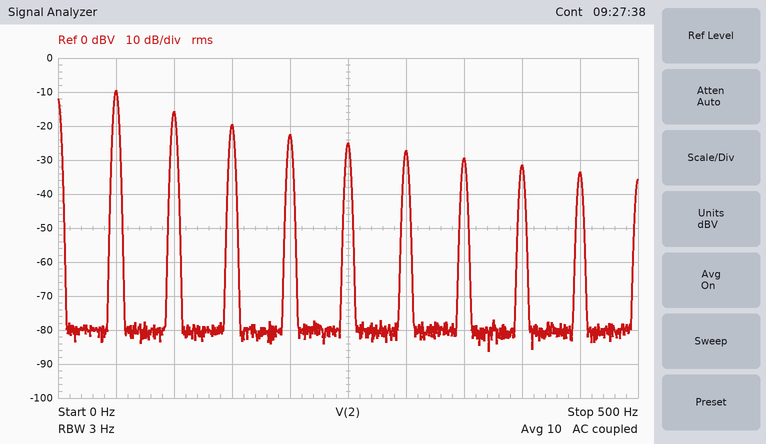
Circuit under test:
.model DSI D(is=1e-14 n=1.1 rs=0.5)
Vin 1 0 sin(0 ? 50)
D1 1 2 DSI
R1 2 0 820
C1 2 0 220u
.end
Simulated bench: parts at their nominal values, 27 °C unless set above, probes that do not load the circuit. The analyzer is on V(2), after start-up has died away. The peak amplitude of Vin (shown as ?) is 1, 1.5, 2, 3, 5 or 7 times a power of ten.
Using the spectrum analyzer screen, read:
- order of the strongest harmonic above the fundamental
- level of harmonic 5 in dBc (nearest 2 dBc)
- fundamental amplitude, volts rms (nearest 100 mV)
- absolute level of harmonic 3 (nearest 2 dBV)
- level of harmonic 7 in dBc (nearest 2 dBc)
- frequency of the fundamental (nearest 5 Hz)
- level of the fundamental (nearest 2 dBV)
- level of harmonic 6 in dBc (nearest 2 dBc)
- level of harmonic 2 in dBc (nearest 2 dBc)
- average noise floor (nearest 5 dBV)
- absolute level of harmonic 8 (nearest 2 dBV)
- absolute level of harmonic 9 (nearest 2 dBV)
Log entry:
2
-16 dBc
300 mV
-20 dBV
-20 dBc
50 Hz
-10 dBV
-18 dBc
-6 dBc
-80 dBV
-32 dBV
-34 dBV
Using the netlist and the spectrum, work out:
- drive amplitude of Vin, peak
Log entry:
15 V
